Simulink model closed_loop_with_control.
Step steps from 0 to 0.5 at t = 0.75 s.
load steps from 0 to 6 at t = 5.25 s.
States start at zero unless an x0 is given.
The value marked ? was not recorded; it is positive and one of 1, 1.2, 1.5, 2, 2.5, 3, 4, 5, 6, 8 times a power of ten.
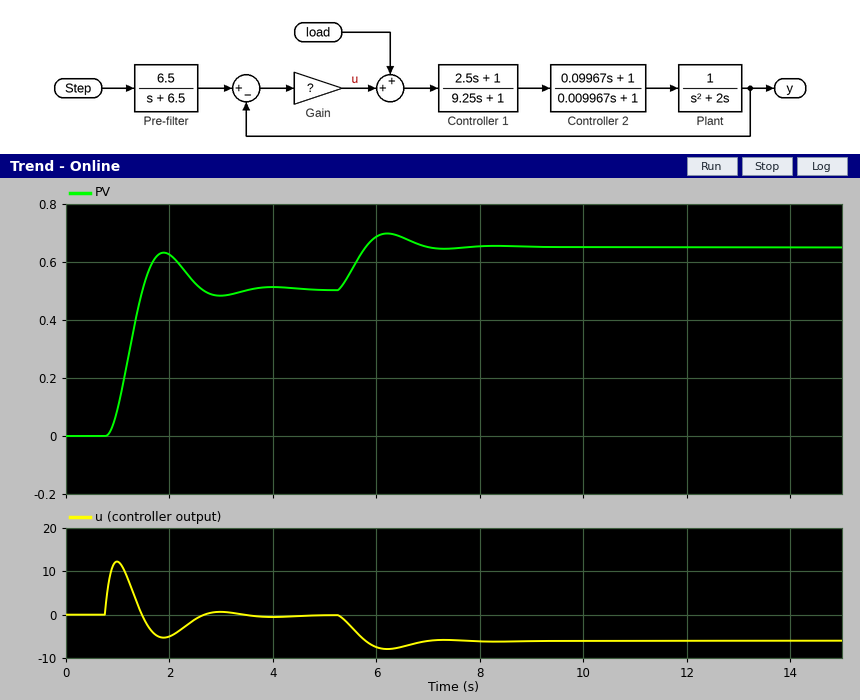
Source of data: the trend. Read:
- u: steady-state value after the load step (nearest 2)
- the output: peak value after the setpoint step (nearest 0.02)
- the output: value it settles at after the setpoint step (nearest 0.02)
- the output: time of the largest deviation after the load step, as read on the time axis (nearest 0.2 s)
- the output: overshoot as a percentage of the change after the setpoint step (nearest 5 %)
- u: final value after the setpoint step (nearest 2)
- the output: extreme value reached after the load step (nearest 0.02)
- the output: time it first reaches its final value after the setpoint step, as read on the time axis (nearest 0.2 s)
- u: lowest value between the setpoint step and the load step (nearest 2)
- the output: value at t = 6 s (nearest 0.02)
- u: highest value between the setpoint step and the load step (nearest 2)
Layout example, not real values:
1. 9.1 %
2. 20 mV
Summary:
1. -6
2. 0.64
3. 0.50
4. 6.2 s
5. 25 %
6. 0
7. 0.70
8. 1.4 s
9. -6
10. 0.68
11. 12
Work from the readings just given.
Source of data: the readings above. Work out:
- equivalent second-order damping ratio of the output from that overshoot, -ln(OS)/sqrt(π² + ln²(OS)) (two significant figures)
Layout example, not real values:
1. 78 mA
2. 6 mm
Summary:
1. 0.40
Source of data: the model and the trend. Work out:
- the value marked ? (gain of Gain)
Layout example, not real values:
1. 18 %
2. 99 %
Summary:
1. 40
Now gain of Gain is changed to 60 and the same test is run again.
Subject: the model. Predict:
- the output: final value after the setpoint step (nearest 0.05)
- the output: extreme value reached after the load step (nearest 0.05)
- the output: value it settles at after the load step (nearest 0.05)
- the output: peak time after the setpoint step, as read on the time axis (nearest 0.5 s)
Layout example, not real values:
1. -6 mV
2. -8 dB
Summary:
1. 0.50
2. 0.65
3. 0.60
4. 1.5 s
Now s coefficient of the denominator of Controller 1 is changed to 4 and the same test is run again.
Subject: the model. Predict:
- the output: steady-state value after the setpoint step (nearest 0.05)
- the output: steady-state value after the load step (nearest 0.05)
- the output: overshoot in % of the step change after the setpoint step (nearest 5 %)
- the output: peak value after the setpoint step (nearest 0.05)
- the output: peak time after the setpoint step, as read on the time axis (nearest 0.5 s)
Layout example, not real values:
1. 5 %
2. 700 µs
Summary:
1. 0.50
2. 0.65
3. 20 %
4. 0.60
5. 1.5 s
